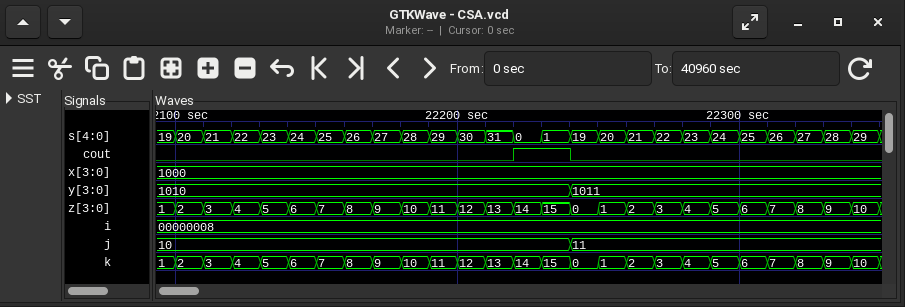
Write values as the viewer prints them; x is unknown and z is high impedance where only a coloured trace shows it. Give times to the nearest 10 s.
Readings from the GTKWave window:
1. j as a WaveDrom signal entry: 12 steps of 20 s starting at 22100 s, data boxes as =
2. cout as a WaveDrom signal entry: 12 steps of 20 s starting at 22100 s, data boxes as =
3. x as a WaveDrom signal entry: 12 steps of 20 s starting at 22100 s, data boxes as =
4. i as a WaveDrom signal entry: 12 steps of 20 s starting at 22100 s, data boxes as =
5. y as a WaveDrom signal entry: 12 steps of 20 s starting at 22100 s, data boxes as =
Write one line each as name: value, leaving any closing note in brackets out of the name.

j as a WaveDrom signal entry: 12 steps of 20 s starting at 22100 s, data boxes as =: {name: 'j', wave: '=......=....', data: '10 11'}
cout as a WaveDrom signal entry: 12 steps of 20 s starting at 22100 s, data boxes as =: {name: 'cout', wave: '0.....10....'}
x as a WaveDrom signal entry: 12 steps of 20 s starting at 22100 s, data boxes as =: {name: 'x', wave: '=...........', data: '1000'}
i as a WaveDrom signal entry: 12 steps of 20 s starting at 22100 s, data boxes as =: {name: 'i', wave: '=...........', data: '00000008'}
y as a WaveDrom signal entry: 12 steps of 20 s starting at 22100 s, data boxes as =: {name: 'y', wave: '=......=....', data: '1010 1011'}
